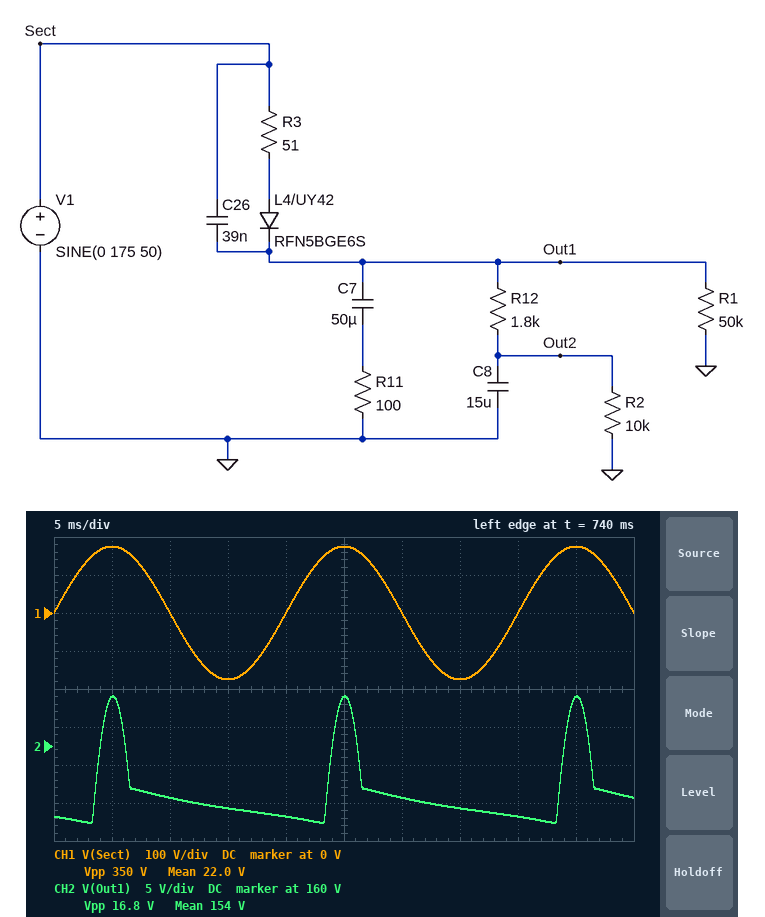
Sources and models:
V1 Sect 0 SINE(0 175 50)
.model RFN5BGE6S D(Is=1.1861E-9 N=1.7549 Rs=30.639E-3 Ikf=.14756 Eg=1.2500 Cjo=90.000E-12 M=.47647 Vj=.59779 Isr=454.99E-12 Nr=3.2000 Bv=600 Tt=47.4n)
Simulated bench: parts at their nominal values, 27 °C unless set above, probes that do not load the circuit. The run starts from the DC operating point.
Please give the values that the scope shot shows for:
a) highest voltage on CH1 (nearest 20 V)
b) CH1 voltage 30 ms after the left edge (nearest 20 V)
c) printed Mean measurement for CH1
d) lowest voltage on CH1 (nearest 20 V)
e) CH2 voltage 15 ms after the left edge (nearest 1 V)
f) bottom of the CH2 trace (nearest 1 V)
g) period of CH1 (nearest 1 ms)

180 V
0 V
22.0 V
-180 V
152 V
150 V
20 ms
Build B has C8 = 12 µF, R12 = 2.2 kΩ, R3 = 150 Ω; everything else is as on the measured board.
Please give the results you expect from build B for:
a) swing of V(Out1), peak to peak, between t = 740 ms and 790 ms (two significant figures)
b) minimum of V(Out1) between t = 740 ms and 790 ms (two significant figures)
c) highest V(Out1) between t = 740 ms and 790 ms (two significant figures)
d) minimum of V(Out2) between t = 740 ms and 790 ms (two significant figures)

14 V
140 V
160 V
120 V
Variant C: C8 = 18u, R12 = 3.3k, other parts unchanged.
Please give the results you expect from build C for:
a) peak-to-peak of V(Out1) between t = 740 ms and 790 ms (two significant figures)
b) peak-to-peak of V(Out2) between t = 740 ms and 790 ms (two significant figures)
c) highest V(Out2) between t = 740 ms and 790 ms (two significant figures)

16 V
440 mV
120 V
